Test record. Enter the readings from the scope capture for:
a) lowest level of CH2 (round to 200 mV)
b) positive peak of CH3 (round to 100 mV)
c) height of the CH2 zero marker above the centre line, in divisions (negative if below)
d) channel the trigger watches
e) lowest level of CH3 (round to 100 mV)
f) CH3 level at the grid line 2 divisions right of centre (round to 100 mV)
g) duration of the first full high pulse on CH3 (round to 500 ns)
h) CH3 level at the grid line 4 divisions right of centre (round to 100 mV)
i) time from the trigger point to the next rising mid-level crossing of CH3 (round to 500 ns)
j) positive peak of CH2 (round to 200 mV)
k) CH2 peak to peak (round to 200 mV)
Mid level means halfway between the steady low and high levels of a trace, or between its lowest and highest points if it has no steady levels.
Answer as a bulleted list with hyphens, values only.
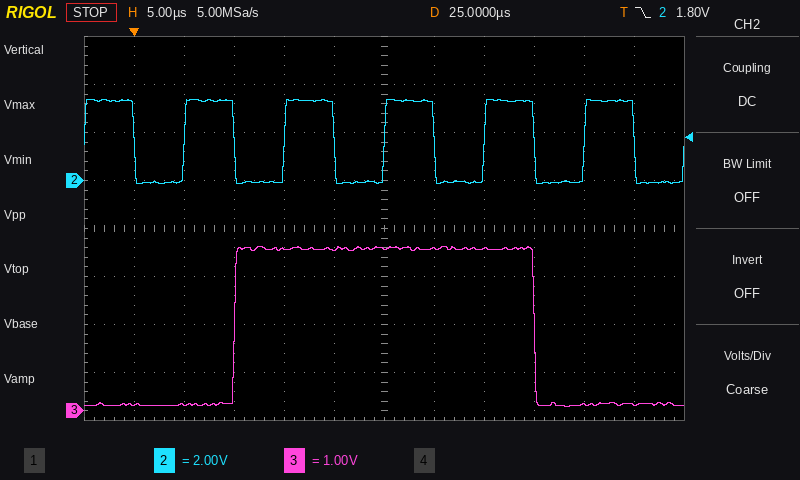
- -200 mV
- 3.4 V
- +1.0 div
- CH2
- 100 mV
- 3.4 V
- 30.0 µs
- 100 mV
- 10.0 µs
- 3.4 V
- 3.6 V
